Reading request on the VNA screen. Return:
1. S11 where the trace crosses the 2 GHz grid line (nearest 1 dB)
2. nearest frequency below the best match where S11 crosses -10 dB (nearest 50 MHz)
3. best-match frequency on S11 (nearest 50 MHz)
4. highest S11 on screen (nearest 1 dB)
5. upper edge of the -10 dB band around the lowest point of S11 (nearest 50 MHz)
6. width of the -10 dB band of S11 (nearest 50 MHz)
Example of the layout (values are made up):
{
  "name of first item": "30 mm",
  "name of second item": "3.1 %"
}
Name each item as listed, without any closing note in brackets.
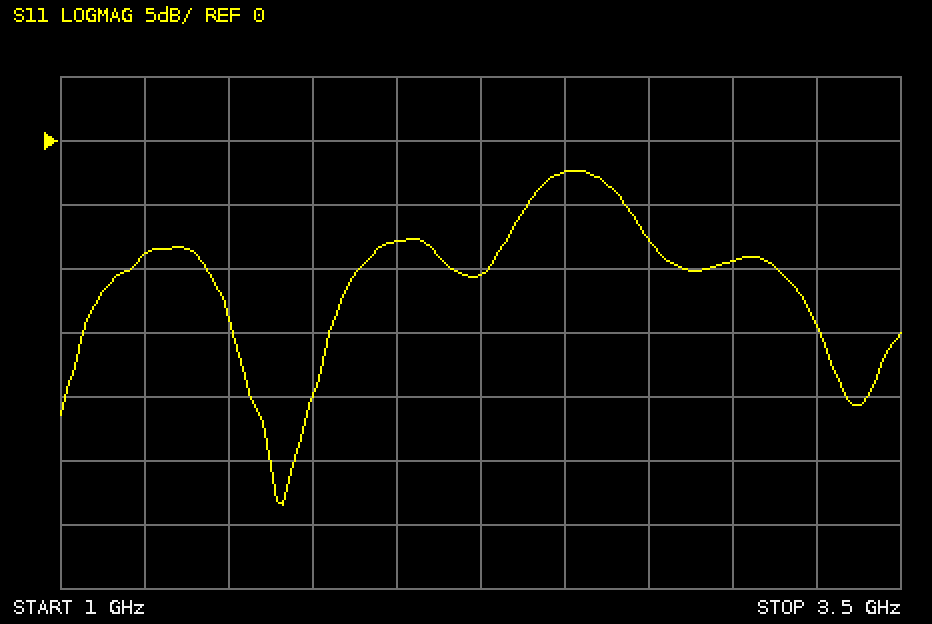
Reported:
{
  "S11 where the trace crosses the 2 GHz grid line": "-8 dB",
  "nearest frequency below the best match where S11 crosses -10 dB": "1.45 GHz",
  "best-match frequency on S11": "1.65 GHz",
  "highest S11 on screen": "-2 dB",
  "upper edge of the -10 dB band around the lowest point of S11": "1.90 GHz",
  "width of the -10 dB band of S11": "450 MHz"
}
